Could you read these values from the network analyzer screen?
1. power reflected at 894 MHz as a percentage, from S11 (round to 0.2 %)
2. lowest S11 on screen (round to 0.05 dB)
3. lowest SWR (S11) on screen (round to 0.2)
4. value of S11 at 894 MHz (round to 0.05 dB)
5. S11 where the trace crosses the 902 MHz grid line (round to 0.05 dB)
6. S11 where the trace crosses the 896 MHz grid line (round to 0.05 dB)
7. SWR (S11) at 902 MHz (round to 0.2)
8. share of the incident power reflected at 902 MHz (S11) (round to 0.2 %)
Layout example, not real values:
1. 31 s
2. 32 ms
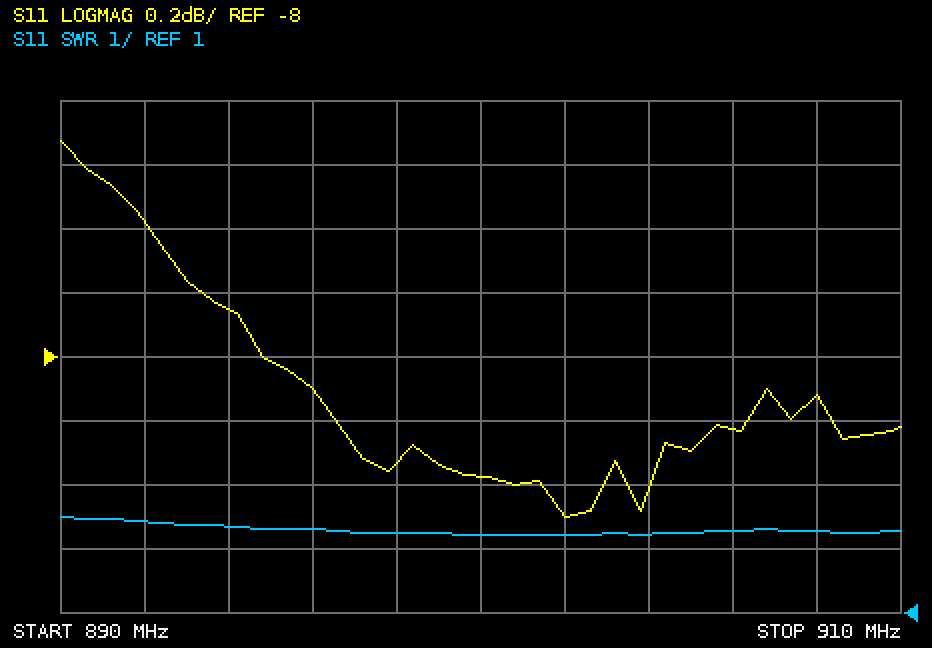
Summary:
1. 16.4 %
2. -8.50 dB
3. 2.2
4. -7.85 dB
5. -8.50 dB
6. -8.10 dB
7. 2.2
8. 14.2 %
